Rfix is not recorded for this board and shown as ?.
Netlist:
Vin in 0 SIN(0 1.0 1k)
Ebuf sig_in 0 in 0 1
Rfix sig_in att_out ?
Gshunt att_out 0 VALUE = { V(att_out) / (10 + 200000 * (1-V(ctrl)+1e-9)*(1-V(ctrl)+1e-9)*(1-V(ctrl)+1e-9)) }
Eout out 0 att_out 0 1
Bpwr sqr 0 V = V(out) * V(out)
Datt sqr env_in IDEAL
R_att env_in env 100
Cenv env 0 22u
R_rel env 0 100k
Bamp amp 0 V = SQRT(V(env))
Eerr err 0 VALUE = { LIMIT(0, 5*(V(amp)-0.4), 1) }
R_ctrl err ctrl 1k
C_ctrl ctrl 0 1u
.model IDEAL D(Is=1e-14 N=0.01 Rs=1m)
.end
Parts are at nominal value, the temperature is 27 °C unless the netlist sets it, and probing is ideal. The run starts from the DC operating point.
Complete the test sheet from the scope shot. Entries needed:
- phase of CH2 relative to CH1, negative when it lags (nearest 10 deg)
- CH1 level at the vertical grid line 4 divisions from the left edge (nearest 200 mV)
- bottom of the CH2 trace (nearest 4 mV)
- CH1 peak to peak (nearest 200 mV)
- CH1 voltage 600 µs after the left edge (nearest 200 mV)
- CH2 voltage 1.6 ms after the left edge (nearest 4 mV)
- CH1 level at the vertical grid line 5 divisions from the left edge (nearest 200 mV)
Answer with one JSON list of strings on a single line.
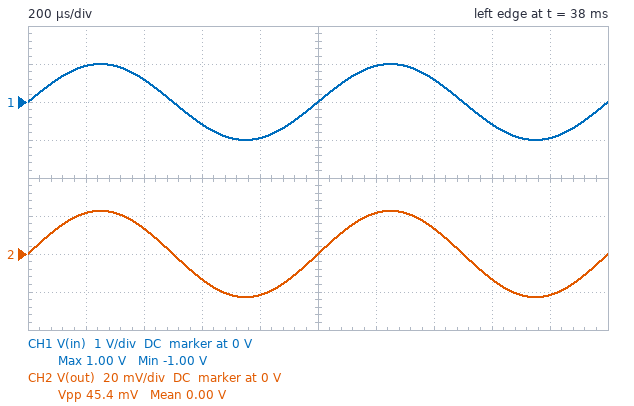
["0 deg", "-1.0 V", "-24 mV", "2.0 V", "-600 mV", "-12 mV", "0 V"]
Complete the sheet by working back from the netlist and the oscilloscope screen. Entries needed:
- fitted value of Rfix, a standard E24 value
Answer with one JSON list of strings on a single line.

["430 Ω"]
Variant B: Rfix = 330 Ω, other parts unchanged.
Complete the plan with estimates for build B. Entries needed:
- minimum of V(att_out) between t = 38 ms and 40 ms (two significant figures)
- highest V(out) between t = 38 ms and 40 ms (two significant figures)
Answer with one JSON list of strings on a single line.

["-29 mV", "29 mV"]
